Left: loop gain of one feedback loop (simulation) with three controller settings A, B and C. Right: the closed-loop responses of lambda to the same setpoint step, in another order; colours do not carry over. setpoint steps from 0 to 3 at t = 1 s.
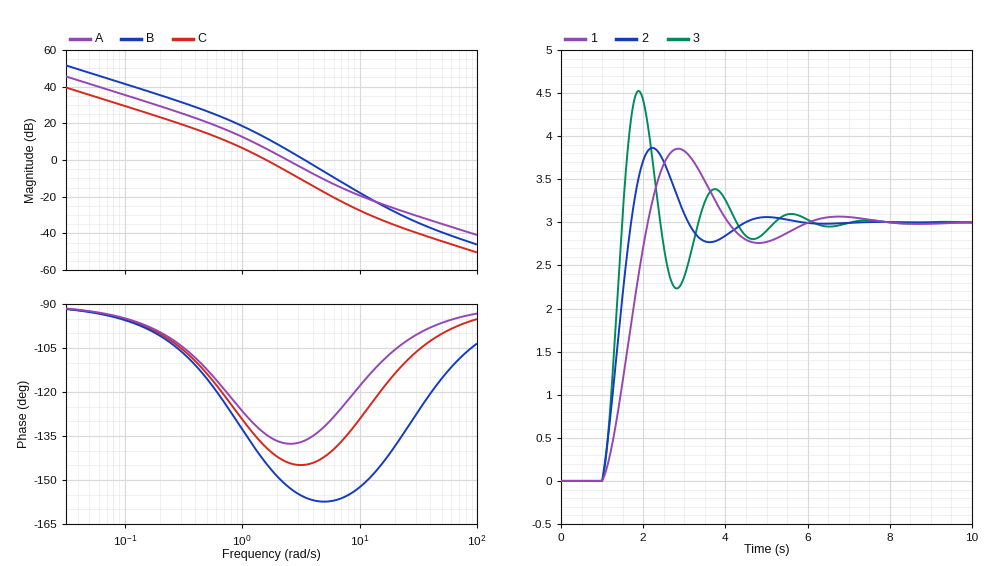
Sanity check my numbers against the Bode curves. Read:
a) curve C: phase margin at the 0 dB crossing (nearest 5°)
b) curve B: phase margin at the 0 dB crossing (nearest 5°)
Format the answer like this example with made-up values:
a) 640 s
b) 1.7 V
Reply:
a) 40°
b) 25°
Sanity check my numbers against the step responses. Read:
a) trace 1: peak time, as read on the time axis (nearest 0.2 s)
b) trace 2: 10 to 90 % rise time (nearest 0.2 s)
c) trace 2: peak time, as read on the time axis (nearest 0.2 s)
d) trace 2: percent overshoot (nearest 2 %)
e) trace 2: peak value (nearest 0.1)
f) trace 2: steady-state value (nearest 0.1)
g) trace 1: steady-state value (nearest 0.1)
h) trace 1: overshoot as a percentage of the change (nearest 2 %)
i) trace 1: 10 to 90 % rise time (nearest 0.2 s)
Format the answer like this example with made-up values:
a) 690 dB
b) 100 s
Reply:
a) 2.8 s
b) 0.6 s
c) 2.2 s
d) 28 %
e) 3.9
f) 3.0
g) 3.0
h) 28 %
i) 0.8 s
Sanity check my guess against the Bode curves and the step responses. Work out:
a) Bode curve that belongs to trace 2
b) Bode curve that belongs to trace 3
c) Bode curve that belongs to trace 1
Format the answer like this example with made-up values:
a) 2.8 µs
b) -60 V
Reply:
a) A
b) B
c) C
